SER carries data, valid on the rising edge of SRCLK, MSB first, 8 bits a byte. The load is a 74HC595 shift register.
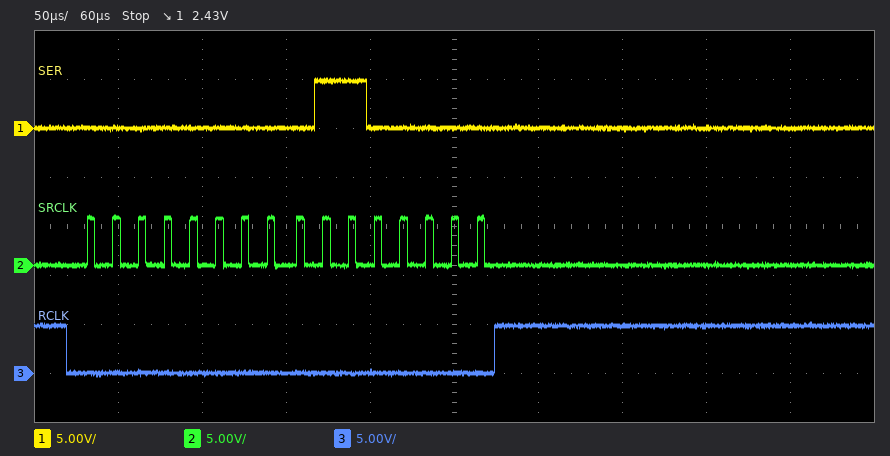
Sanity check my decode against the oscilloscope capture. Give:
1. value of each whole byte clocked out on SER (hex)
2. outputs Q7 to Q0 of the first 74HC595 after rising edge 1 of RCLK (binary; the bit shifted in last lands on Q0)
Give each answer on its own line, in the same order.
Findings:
0x00 0x60
01100000
